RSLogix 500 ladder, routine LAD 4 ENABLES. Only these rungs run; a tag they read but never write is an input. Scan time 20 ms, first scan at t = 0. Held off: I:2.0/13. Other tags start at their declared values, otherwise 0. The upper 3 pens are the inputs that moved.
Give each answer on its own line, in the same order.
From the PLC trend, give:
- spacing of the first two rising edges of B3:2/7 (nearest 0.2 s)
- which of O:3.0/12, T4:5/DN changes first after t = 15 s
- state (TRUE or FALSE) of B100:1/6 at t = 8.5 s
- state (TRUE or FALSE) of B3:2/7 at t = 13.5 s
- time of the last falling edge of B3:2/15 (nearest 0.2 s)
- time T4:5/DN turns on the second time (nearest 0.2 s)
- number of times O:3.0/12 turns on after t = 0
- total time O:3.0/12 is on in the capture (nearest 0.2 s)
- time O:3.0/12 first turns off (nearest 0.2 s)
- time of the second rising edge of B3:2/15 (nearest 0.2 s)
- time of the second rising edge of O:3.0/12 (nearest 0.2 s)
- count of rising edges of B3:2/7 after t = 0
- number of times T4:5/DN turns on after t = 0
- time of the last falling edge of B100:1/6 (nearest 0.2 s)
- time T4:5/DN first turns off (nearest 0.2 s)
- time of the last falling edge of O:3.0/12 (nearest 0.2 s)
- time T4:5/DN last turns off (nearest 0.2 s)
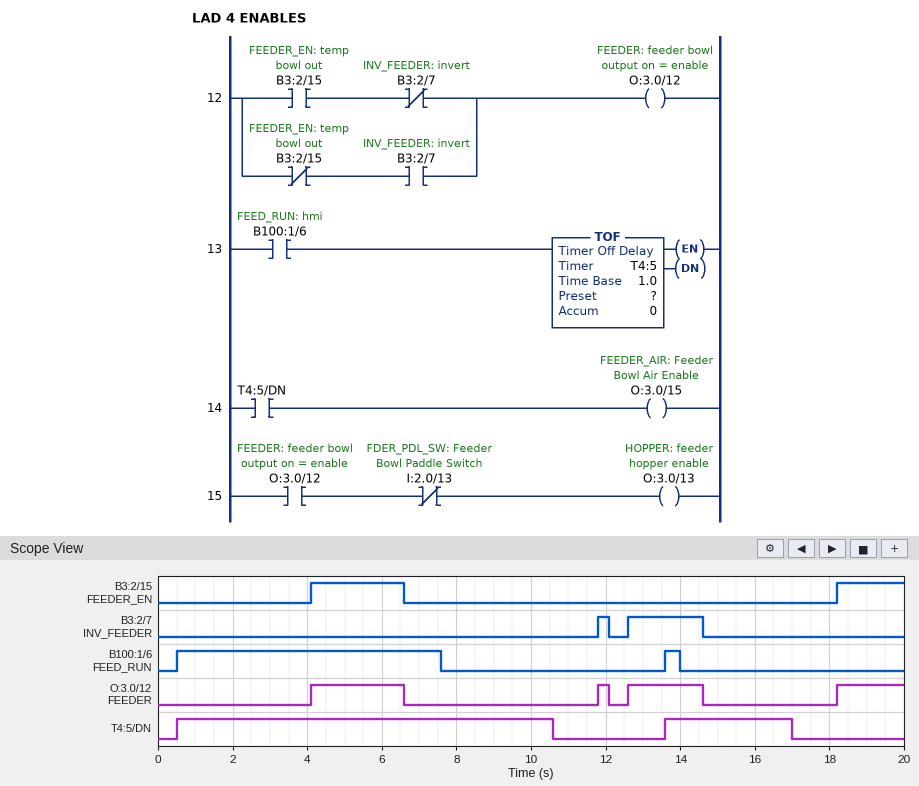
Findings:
0.8 s
T4:5/DN
FALSE
TRUE
6.6 s
13.6 s
4
6.6 s
6.6 s
18.2 s
11.8 s
2
2
14.0 s
10.6 s
14.6 s
17.0 s
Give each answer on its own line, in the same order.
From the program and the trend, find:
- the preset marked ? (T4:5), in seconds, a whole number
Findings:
3 s
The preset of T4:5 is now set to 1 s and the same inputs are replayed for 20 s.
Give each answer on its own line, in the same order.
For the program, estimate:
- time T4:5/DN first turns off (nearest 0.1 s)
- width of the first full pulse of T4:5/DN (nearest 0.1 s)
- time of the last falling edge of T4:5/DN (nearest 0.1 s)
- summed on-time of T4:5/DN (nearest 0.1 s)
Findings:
8.6 s
8.1 s
15.0 s
9.5 s
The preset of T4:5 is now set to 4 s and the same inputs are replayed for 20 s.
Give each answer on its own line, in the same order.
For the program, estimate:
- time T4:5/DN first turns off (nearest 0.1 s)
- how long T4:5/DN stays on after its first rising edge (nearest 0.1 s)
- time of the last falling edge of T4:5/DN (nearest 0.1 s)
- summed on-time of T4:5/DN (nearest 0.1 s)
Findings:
11.6 s
11.1 s
18.0 s
15.5 s
